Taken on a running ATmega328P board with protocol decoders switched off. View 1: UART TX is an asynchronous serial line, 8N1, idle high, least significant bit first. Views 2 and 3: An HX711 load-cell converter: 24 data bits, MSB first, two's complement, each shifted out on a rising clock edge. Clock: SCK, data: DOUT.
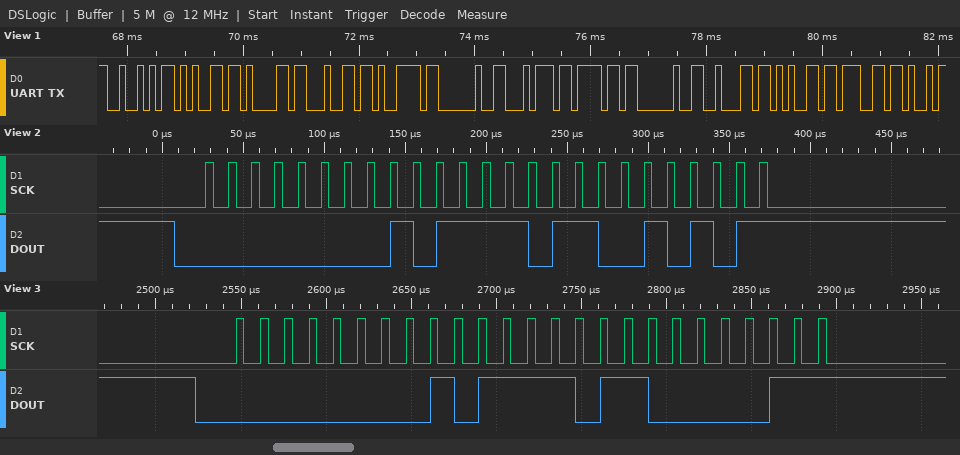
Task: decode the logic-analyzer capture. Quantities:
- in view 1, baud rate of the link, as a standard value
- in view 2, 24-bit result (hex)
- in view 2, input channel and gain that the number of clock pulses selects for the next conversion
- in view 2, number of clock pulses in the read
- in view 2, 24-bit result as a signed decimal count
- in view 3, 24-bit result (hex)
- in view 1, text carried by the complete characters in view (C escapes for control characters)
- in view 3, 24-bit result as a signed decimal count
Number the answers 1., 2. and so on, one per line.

1. 9600 baud
2. 0x00BD95
3. channel A, gain 128
4. 25
5. 48533
6. 0x00BD83
7. "Ready to beg"
8. 48515
